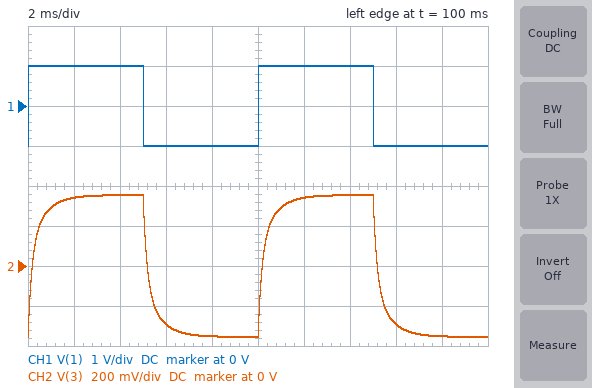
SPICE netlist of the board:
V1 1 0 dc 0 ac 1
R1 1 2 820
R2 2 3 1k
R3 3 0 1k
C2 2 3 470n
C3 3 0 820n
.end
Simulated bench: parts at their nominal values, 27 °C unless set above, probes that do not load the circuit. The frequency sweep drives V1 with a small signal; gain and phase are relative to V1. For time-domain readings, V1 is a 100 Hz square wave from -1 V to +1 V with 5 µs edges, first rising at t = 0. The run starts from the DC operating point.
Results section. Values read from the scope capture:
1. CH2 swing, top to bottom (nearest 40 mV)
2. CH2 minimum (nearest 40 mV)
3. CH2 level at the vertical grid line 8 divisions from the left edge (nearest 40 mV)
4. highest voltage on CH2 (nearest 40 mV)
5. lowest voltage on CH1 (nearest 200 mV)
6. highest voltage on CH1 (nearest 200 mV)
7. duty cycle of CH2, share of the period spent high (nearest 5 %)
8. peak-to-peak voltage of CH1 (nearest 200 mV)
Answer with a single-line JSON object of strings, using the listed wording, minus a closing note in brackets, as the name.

{"CH2 swing, top to bottom": "720 mV", "CH2 minimum": "-360 mV", "CH2 level at the vertical grid line 8 divisions from the left edge": "-280 mV", "highest voltage on CH2": "360 mV", "lowest voltage on CH1": "-1.0 V", "highest voltage on CH1": "1.0 V", "duty cycle of CH2, share of the period spent high": "50 %", "peak-to-peak voltage of CH1": "2.0 V"}
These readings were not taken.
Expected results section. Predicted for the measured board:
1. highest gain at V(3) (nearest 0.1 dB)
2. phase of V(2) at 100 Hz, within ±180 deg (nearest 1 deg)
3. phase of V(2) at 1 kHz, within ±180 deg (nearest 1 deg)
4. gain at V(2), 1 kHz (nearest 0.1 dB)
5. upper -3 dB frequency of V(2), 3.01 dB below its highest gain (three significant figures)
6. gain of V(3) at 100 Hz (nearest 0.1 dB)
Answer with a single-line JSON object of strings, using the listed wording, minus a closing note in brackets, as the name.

{"highest gain at V(3)": "-9.0 dB", "phase of V(2) at 100 Hz, within ±180 deg": "-7 deg", "phase of V(2) at 1 kHz, within ±180 deg": "-47 deg", "gain at V(2), 1 kHz": "-6.5 dB", "upper -3 dB frequency of V(2), 3.01 dB below its highest gain": "892 Hz", "gain of V(3) at 100 Hz": "-9.4 dB"}
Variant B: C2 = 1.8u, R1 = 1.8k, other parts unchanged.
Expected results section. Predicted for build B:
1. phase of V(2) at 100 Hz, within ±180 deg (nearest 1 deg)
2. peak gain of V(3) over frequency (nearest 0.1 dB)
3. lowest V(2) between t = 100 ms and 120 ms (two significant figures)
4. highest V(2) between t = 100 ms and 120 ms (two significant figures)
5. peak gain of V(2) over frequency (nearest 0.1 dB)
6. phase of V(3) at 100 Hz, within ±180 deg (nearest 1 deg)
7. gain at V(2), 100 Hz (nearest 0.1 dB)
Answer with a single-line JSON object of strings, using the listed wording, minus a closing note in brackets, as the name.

{"phase of V(2) at 100 Hz, within ±180 deg": "-20 deg", "peak gain of V(3) over frequency": "-11.0 dB", "lowest V(2) between t = 100 ms and 120 ms": "-520 mV", "highest V(2) between t = 100 ms and 120 ms": "520 mV", "peak gain of V(2) over frequency": "-5.6 dB", "phase of V(3) at 100 Hz, within ±180 deg": "-11 deg", "gain at V(2), 100 Hz": "-6.3 dB"}
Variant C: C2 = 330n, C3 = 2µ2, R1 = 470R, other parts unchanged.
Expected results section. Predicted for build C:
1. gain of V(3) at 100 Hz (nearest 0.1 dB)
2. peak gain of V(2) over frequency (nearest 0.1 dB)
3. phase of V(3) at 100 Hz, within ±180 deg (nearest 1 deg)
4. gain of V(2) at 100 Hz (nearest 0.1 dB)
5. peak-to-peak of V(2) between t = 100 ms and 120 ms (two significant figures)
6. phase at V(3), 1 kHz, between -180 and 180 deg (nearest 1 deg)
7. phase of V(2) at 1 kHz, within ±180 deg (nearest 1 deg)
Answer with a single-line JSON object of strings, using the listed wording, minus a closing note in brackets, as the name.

{"gain of V(3) at 100 Hz": "-10.2 dB", "peak gain of V(2) over frequency": "-1.8 dB", "phase of V(3) at 100 Hz, within ±180 deg": "-33 deg", "gain of V(2) at 100 Hz": "-2.2 dB", "peak-to-peak of V(2) between t = 100 ms and 120 ms": "1.6 V", "phase at V(3), 1 kHz, between -180 and 180 deg": "-51 deg", "phase of V(2) at 1 kHz, within ±180 deg": "-32 deg"}
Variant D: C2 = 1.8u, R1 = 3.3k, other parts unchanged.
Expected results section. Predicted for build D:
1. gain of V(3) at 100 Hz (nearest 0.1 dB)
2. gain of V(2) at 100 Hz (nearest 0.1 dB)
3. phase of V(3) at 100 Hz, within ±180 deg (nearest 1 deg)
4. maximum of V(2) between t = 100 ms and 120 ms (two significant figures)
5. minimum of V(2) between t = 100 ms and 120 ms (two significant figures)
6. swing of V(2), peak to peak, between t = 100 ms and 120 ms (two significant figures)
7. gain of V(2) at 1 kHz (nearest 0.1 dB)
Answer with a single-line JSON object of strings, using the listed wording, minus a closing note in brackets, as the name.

{"gain of V(3) at 100 Hz": "-14.3 dB", "gain of V(2) at 100 Hz": "-9.6 dB", "phase of V(3) at 100 Hz, within ±180 deg": "-16 deg", "maximum of V(2) between t = 100 ms and 120 ms": "370 mV", "minimum of V(2) between t = 100 ms and 120 ms": "-370 mV", "swing of V(2), peak to peak, between t = 100 ms and 120 ms": "740 mV", "gain of V(2) at 1 kHz": "-21.6 dB"}
